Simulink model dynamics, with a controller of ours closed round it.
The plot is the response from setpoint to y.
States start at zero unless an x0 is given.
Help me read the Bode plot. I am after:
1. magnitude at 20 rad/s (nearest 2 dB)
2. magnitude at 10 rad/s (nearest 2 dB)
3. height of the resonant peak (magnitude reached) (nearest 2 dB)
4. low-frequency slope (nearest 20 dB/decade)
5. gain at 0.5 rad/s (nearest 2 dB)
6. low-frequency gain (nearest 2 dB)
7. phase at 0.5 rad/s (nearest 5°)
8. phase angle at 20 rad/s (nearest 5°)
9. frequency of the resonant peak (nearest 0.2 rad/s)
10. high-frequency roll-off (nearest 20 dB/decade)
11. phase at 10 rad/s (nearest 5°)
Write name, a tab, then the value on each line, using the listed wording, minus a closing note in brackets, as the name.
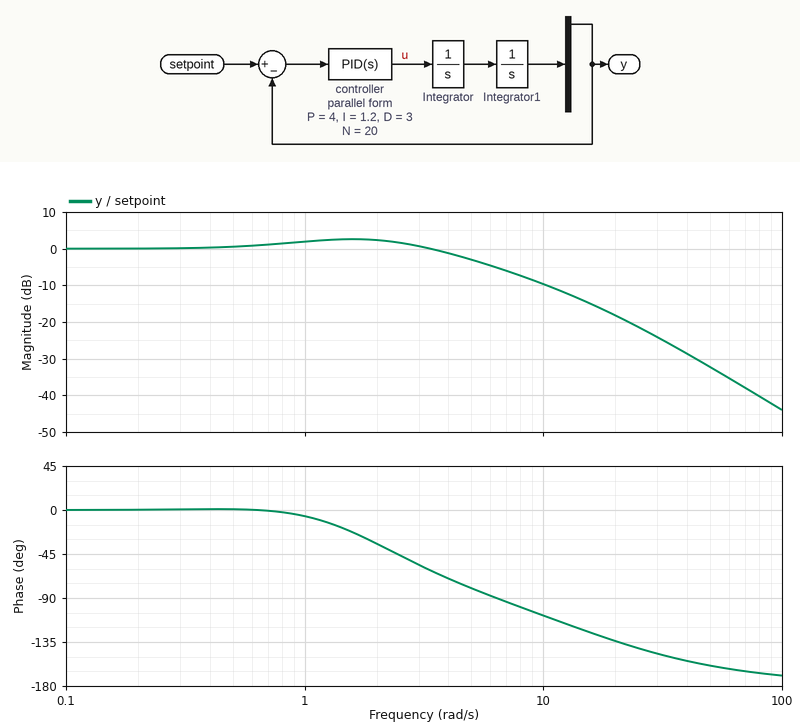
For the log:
magnitude at 20 rad/s	-18 dB
magnitude at 10 rad/s	-10 dB
height of the resonant peak (magnitude reached)	2 dB
low-frequency slope	0 dB/decade
gain at 0.5 rad/s	0 dB
low-frequency gain	0 dB
phase at 0.5 rad/s	0°
phase angle at 20 rad/s	-135°
frequency of the resonant peak	1.6 rad/s
high-frequency roll-off	-40 dB/decade
phase at 10 rad/s	-110°
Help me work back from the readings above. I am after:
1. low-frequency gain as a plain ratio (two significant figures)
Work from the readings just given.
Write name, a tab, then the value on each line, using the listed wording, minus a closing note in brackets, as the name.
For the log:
low-frequency gain as a plain ratio	1.0
